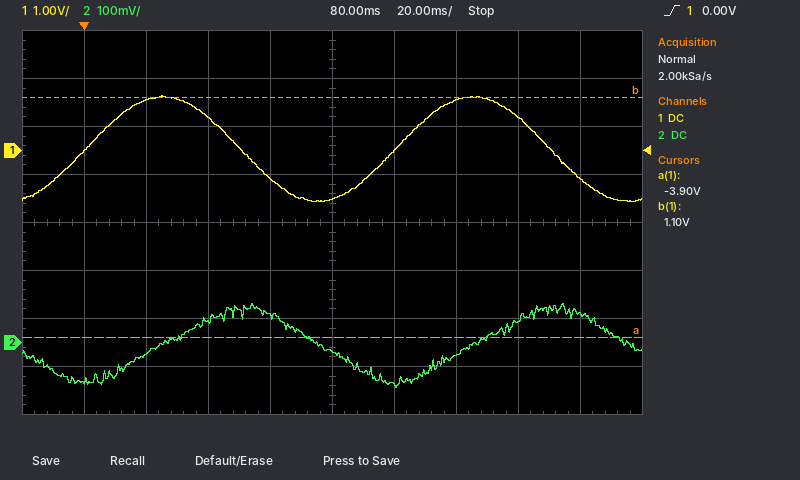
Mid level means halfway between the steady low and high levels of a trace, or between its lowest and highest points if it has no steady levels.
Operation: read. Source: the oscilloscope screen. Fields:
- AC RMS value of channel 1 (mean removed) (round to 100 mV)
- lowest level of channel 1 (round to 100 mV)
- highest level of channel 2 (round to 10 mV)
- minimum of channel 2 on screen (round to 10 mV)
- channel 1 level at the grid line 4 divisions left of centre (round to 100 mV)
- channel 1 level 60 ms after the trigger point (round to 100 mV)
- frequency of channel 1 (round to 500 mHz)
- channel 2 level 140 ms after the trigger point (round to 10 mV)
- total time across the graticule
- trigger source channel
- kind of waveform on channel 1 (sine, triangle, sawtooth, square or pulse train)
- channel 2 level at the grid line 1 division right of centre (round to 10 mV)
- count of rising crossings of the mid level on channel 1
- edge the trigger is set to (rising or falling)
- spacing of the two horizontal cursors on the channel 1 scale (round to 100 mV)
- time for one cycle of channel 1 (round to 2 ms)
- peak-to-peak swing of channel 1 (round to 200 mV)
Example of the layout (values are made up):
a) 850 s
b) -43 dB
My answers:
a) 800 mV
b) -1.1 V
c) 80 mV
d) -90 mV
e) 0.0 V
f) -600 mV
g) 10.0 Hz
h) 50 mV
i) 200 ms
j) channel 1
k) sine
l) -90 mV
m) 2
n) rising
o) 5.0 V
p) 100 ms
q) 2.2 V
